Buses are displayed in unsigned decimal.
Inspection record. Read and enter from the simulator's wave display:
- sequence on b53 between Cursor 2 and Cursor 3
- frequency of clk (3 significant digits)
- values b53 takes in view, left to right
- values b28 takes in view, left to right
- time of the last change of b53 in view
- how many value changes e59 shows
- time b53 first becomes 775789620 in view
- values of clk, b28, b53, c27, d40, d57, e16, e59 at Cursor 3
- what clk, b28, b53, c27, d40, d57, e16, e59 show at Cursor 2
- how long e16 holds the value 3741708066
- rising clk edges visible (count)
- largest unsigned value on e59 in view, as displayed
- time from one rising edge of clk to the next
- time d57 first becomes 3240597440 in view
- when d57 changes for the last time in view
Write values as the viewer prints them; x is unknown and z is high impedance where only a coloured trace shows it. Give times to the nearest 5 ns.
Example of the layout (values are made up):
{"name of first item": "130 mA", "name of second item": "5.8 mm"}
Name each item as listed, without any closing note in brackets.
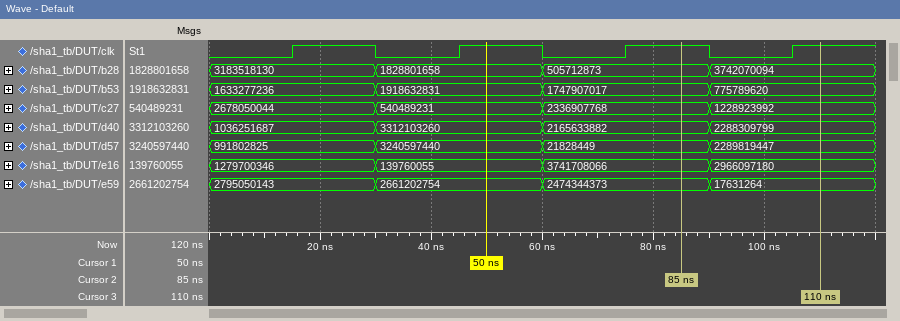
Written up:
{"sequence on b53 between Cursor 2 and Cursor 3": "1747907017, 775789620", "frequency of clk": "33.3 MHz", "values b53 takes in view, left to right": "1633277236, 1918632831, 1747907017, 775789620", "values b28 takes in view, left to right": "3183518130, 1828801658, 505712873, 3742070094", "time of the last change of b53 in view": "90 ns", "how many value changes e59 shows": "3", "time b53 first becomes 775789620 in view": "90 ns", "values of clk, b28, b53, c27, d40, d57, e16, e59 at Cursor 3": "clk=1, b28=3742070094, b53=775789620, c27=1228923992, d40=2288309799, d57=2289819447, e16=2966097180, e59=17631264", "what clk, b28, b53, c27, d40, d57, e16, e59 show at Cursor 2": "clk=1, b28=505712873, b53=1747907017, c27=2336907768, d40=2165633882, d57=21828449, e16=3741708066, e59=2474344373", "how long e16 holds the value 3741708066": "30 ns", "rising clk edges visible": "4", "largest unsigned value on e59 in view, as displayed": "2795050143", "time from one rising edge of clk to the next": "30 ns", "time d57 first becomes 3240597440 in view": "30 ns", "when d57 changes for the last time in view": "90 ns"}
